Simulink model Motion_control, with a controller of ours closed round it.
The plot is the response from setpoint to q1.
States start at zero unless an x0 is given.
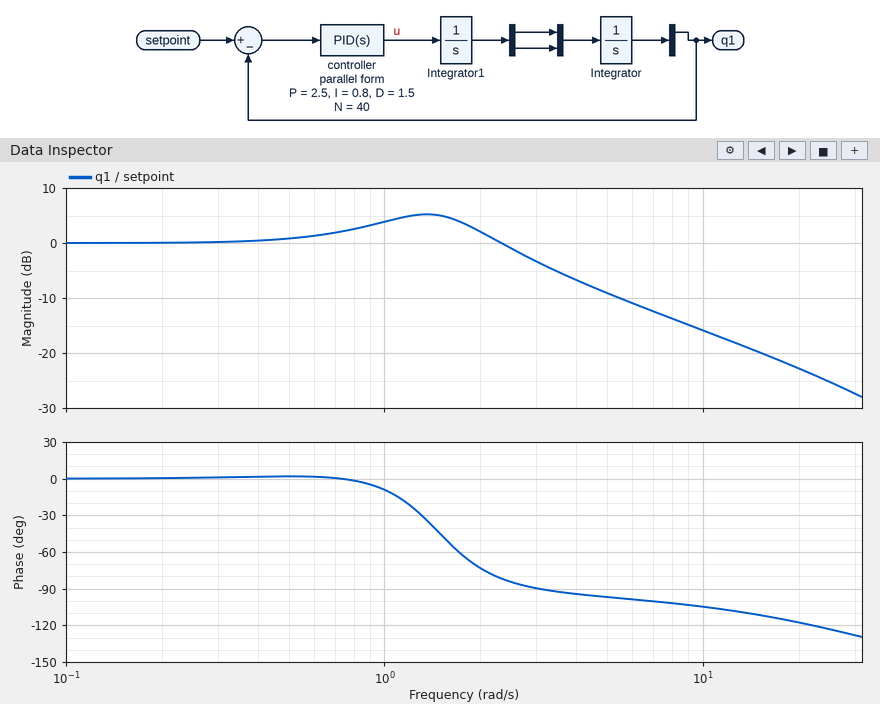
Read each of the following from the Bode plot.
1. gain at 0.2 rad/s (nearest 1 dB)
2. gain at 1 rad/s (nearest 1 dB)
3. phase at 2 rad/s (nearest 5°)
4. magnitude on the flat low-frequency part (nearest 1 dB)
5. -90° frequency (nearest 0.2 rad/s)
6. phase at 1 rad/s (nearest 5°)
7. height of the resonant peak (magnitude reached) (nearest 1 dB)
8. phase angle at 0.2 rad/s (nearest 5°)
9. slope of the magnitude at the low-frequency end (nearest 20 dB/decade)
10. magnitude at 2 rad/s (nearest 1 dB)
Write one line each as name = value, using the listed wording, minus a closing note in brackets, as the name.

gain at 0.2 rad/s = 0 dB
gain at 1 rad/s = 4 dB
phase at 2 rad/s = -75°
magnitude on the flat low-frequency part = 0 dB
-90° frequency = 3.0 rad/s
phase at 1 rad/s = -10°
height of the resonant peak (magnitude reached) = 5 dB
phase angle at 0.2 rad/s = 0°
slope of the magnitude at the low-frequency end = 0 dB/decade
magnitude at 2 rad/s = 2 dB
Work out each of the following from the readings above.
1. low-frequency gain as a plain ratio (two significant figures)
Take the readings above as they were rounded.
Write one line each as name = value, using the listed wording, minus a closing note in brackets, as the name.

low-frequency gain as a plain ratio = 1.0
